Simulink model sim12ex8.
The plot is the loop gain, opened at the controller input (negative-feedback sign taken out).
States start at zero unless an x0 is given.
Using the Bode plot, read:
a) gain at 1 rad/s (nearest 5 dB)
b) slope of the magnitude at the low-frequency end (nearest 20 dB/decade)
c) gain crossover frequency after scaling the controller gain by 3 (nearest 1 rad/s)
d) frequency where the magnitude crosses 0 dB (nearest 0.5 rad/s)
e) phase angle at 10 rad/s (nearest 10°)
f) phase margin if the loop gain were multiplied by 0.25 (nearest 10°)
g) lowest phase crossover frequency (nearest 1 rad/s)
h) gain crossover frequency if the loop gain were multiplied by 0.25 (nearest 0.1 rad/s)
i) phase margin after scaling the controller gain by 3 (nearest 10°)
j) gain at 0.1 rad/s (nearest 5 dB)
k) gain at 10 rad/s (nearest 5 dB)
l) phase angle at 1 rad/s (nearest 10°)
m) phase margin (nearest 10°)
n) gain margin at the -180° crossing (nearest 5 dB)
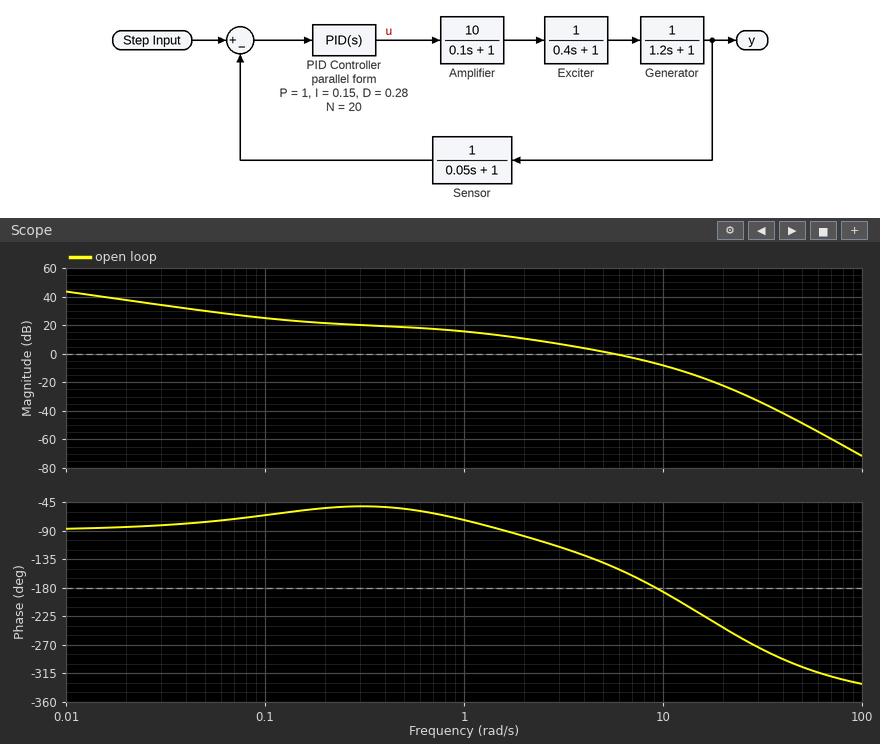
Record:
15 dB
-20 dB/decade
11 rad/s
5.5 rad/s
-190°
90°
9 rad/s
1.7 rad/s
-10°
25 dB
-10 dB
-70°
30°
5 dB
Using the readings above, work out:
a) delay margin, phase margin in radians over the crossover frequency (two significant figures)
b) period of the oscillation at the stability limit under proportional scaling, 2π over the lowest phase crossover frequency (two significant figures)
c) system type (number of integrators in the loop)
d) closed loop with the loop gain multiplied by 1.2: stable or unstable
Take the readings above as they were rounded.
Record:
0.095 s
0.70 s
1
stable
